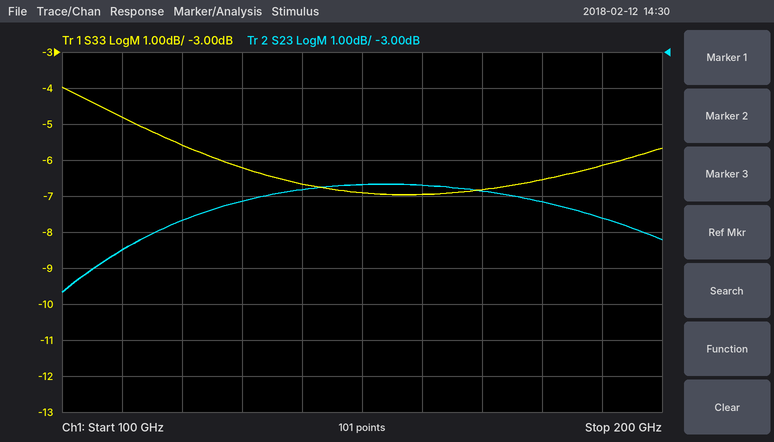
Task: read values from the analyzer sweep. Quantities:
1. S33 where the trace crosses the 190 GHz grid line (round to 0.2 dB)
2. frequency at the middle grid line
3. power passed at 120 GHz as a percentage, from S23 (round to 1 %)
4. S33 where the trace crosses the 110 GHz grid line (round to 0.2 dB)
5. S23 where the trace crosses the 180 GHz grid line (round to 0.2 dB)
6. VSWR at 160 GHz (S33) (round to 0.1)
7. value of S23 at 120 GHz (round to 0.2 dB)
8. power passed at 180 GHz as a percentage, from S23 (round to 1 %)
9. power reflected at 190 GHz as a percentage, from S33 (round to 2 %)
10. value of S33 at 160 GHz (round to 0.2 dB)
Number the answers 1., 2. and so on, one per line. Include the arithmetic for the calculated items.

1. -6.2 dB
2. 150 GHz
3. 10^(-7.6/10) ≈ 17 %
4. -4.8 dB
5. -7.2 dB
6. |Γ| = 10^(-7/20) = 0.4467; VSWR = (1 + 0.4467)/(1 − 0.4467) ≈ 2.6
7. -7.6 dB
8. 10^(-7.2/10) ≈ 19 %
9. 10^(-6.2/10) ≈ 24 %
10. -7.0 dB
